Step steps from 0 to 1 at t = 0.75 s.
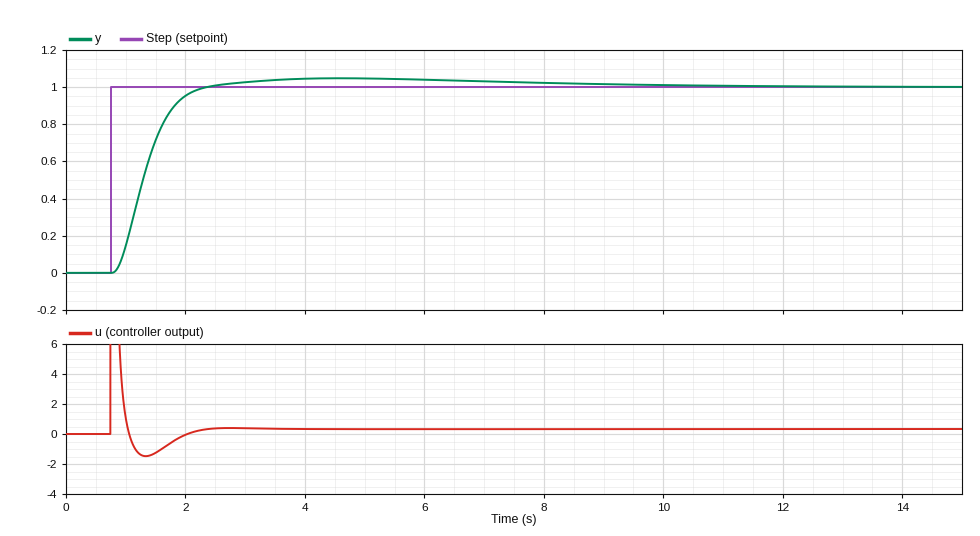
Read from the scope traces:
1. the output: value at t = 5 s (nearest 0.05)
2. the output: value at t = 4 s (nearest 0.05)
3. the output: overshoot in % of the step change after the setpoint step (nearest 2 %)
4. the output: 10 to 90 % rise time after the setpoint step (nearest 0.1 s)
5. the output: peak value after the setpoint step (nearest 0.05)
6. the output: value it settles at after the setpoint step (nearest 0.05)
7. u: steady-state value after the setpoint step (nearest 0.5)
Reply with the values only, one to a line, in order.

1.05
1.05
4 %
0.9 s
1.05
1.00
0.5
